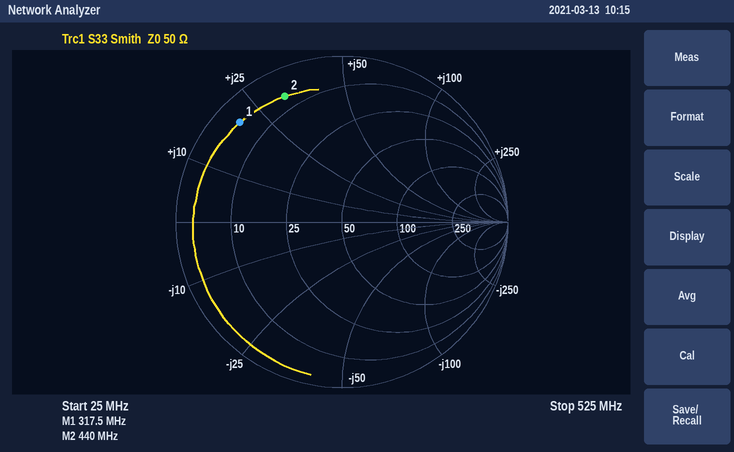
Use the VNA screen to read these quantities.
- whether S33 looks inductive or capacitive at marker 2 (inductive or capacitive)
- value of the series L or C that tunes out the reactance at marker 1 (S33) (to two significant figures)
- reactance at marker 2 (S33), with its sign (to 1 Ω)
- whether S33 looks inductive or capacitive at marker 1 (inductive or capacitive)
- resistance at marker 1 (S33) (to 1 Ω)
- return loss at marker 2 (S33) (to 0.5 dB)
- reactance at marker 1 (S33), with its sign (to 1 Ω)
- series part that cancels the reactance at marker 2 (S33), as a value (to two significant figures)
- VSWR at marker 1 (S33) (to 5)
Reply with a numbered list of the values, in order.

1. inductive
2. 25 pF
3. +32 Ω
4. inductive
5. 4 Ω
6. 1.5 dB
7. +20 Ω
8. 11 pF
9. 15
